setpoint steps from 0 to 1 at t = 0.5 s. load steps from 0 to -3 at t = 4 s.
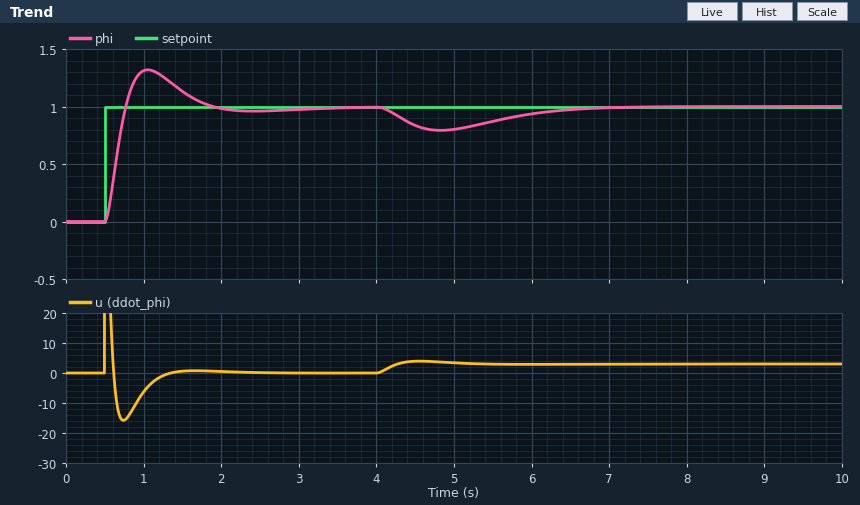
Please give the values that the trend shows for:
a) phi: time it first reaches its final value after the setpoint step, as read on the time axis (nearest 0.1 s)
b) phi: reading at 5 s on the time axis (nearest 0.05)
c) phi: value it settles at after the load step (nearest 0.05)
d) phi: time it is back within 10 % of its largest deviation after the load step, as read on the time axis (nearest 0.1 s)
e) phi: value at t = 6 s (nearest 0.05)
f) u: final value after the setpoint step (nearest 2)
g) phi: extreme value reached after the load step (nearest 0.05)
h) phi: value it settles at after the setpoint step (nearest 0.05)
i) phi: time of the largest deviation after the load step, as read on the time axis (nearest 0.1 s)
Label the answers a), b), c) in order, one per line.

a) 0.8 s
b) 0.80
c) 1.00
d) 6.7 s
e) 0.95
f) 0
g) 0.80
h) 1.00
i) 4.8 s
